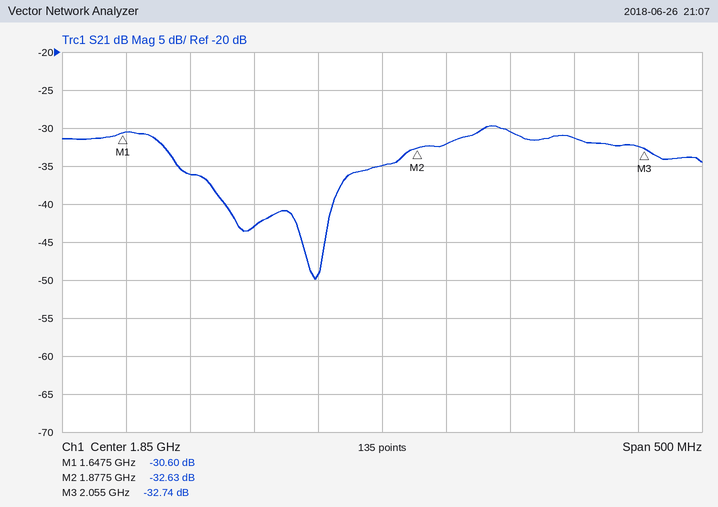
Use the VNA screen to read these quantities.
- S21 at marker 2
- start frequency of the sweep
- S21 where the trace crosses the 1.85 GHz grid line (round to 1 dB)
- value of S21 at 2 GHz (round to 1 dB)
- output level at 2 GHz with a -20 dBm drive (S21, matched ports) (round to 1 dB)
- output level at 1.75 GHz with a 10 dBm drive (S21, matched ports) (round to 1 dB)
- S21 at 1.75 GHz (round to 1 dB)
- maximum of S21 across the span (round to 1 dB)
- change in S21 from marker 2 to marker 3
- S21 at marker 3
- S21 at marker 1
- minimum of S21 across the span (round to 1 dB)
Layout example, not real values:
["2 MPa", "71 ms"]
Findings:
["-32.63 dB", "1.6 GHz", "-35 dB", "-31 dB", "-51 dBm", "-33 dBm", "-43 dB", "-30 dB", "-0.11 dB", "-32.74 dB", "-30.60 dB", "-50 dB"]
